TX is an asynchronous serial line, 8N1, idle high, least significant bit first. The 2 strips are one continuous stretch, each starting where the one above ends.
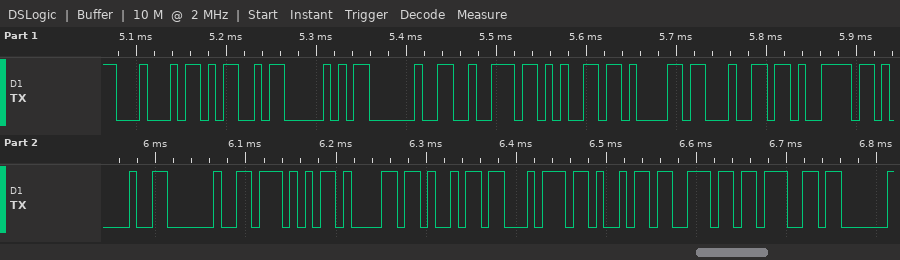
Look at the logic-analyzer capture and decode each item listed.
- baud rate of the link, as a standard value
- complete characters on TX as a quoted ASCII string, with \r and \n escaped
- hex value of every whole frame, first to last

115200 baud
"DMP ready! Waiting"
0x44 0x4D 0x50 0x20 0x72 0x65 0x61 0x64 0x79 0x21 0x20 0x57 0x61 0x69 0x74 0x69 0x6E 0x67
